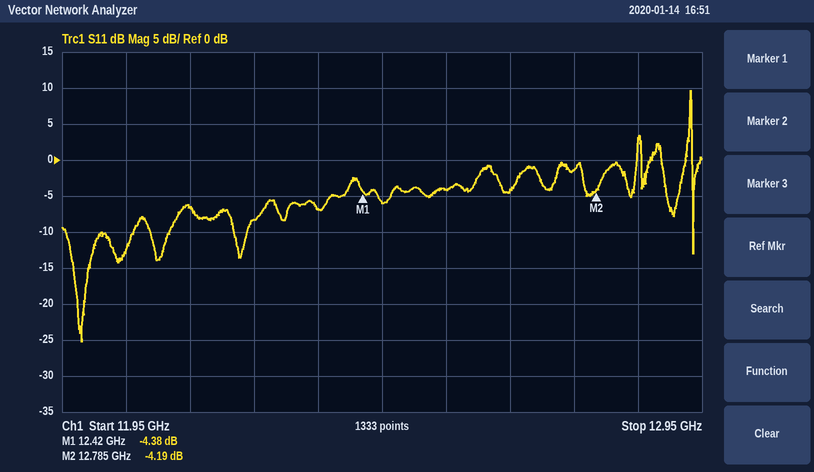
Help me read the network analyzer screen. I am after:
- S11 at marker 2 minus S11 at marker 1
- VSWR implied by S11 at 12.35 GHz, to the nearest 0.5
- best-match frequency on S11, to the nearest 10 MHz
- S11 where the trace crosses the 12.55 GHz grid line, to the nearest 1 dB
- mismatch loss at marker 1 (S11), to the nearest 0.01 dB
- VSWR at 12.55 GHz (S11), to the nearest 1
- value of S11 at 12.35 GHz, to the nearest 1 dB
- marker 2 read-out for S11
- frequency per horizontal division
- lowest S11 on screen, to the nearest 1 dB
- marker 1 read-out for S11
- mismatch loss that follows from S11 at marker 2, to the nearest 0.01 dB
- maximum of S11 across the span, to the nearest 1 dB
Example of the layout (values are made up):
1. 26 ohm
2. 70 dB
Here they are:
1. 0.19 dB
2. 2.5
3. 11.98 GHz
4. -4 dB
5. 1.97 dB
6. 4
7. -7 dB
8. -4.19 dB
9. 100 MHz
10. -25 dB
11. -4.38 dB
12. 2.08 dB
13. 10 dB
